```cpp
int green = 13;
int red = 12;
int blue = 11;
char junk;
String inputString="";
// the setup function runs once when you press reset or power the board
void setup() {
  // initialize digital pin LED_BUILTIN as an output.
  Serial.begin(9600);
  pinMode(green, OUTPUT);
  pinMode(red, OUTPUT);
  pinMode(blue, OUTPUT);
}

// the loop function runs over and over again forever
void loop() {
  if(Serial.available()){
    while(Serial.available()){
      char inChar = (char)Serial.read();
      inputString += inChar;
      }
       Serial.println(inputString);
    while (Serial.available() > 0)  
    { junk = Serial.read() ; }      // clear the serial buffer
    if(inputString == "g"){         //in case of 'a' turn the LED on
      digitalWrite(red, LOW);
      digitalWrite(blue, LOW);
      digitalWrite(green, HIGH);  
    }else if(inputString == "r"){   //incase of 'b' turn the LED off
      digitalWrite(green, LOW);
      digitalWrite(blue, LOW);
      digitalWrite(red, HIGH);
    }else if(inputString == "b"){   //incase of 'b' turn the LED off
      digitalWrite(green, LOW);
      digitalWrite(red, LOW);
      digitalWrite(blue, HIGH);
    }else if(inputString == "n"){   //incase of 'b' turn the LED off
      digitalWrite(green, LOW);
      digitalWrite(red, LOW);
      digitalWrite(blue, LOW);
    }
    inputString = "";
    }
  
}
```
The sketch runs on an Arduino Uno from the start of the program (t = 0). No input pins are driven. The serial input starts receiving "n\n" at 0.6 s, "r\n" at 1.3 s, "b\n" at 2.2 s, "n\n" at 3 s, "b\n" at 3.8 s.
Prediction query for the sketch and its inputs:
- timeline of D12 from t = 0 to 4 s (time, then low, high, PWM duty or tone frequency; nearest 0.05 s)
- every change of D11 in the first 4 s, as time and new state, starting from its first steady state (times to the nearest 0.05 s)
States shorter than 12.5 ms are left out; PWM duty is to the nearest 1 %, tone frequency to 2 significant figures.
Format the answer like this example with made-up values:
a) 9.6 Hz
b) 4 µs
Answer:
a) 0 s low; 1.3 s high; 2.2 s low
b) 0 s low; 2.2 s high; 3 s low; 3.8 s high
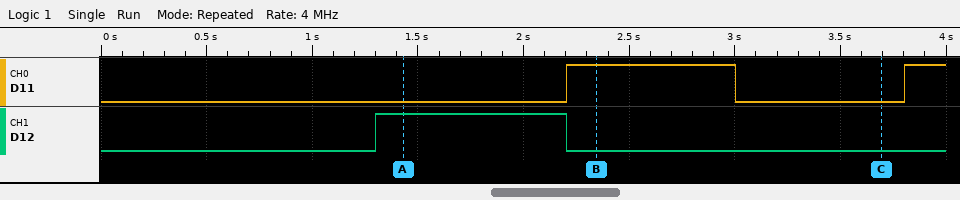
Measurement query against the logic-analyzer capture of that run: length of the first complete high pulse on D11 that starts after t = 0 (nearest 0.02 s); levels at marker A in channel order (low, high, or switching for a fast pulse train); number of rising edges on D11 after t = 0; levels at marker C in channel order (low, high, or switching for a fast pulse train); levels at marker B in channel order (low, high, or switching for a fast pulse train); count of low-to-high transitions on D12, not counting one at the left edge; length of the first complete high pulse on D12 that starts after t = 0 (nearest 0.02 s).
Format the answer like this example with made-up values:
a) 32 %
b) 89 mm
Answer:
a) 0.80 s
b) D11 low, D12 high
c) 2
d) D11 low, D12 low
e) D11 high, D12 low
f) 1
g) 0.90 s
